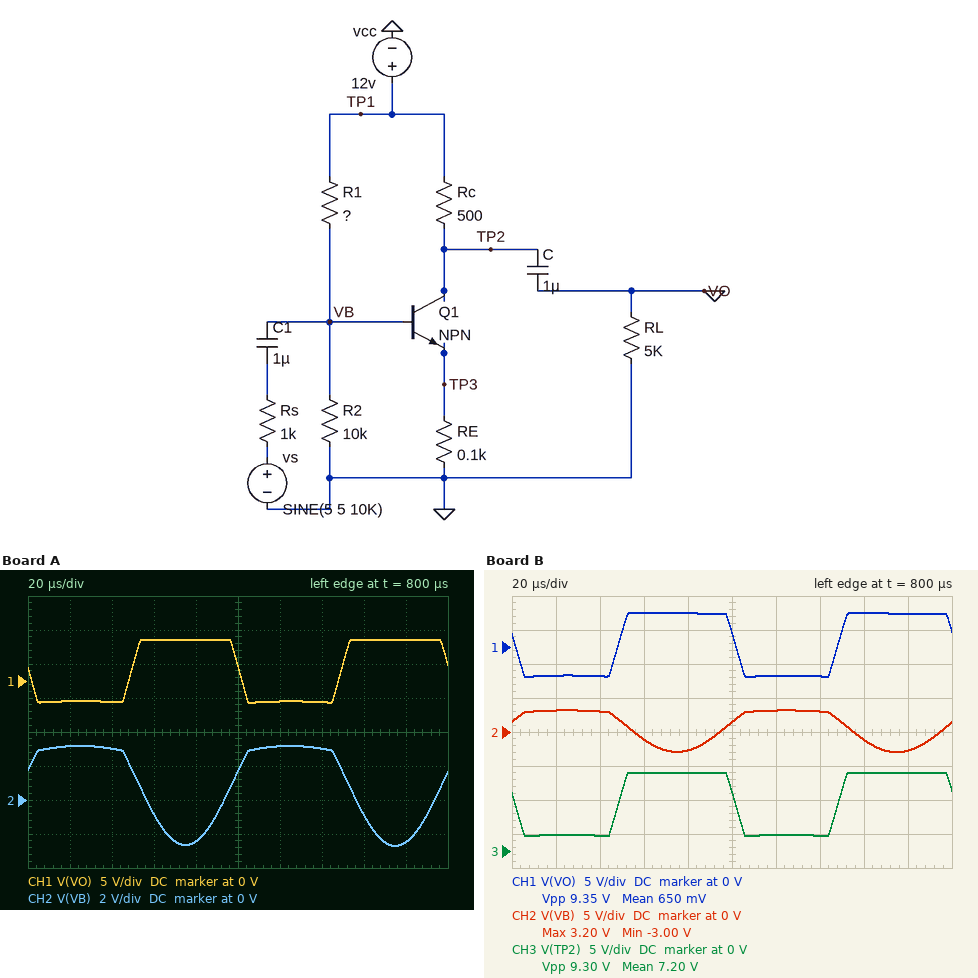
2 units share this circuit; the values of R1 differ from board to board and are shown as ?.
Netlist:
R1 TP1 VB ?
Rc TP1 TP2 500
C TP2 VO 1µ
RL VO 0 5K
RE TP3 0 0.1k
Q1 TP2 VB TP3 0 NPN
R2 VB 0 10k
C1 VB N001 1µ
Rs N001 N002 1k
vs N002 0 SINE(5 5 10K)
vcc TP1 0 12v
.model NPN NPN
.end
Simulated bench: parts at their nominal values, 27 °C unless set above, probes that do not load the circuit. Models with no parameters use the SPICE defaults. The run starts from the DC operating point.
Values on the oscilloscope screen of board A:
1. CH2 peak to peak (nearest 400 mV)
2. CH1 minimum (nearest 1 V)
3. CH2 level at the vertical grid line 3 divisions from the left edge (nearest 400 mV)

6.0 V
-3 V
-800 mV
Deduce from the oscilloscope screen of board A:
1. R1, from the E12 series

27 kΩ
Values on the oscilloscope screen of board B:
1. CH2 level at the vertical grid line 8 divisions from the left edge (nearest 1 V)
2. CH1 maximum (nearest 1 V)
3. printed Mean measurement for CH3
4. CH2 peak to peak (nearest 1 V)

-1 V
5 V
7.20 V
6 V
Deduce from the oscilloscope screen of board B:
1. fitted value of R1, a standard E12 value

33 kΩ
